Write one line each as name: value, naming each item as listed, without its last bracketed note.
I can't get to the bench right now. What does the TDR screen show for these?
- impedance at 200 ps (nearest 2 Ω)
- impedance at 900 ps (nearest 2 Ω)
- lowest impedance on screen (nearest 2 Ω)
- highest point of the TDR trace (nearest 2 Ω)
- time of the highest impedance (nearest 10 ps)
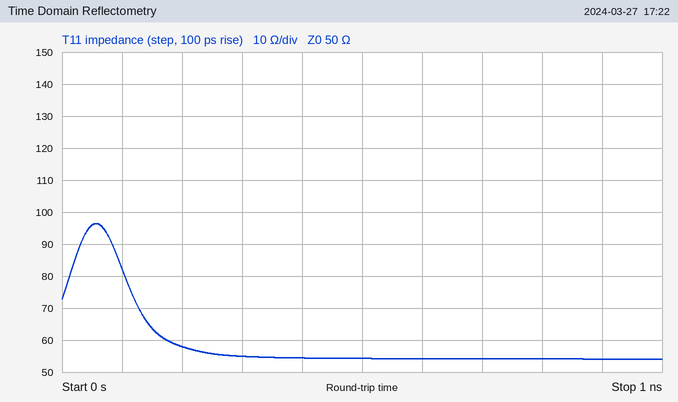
impedance at 200 ps: 58 Ω
impedance at 900 ps: 54 Ω
lowest impedance on screen: 54 Ω
highest point of the TDR trace: 96 Ω
time of the highest impedance: 60 ps
